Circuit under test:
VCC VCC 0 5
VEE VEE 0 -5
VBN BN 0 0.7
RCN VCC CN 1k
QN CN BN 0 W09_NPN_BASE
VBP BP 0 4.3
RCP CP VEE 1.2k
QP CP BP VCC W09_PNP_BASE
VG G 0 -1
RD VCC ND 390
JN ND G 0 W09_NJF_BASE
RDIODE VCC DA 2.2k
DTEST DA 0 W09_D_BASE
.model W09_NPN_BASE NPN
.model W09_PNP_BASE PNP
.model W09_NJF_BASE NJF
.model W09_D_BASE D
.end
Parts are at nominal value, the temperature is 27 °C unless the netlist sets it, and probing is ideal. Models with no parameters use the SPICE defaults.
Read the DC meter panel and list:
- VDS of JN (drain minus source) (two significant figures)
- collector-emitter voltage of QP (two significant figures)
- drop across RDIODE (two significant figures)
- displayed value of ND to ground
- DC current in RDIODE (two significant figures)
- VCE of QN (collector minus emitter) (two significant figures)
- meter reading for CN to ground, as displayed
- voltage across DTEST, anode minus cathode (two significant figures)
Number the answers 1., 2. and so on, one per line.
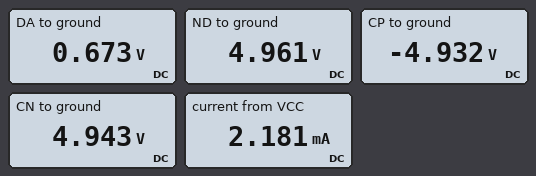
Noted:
1. 5.0 V
2. -9.9 V
3. 4.3 V
4. 4.961 V
5. 2.0 mA
6. 4.9 V
7. 4.943 V
8. 670 mV
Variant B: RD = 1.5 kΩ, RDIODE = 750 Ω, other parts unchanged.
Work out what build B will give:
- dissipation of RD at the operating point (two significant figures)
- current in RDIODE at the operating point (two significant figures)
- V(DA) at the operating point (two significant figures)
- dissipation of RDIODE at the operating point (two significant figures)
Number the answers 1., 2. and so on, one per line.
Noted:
1. 15 µW
2. 5.7 mA
3. 700 mV
4. 25 mW
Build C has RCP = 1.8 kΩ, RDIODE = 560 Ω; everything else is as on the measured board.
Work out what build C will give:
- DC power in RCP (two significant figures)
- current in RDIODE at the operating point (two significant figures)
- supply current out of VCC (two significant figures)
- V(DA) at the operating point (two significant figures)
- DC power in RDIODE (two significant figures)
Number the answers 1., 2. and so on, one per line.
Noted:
1. 5.8 µW
2. 7.7 mA
3. 7.9 mA
4. 710 mV
5. 33 mW
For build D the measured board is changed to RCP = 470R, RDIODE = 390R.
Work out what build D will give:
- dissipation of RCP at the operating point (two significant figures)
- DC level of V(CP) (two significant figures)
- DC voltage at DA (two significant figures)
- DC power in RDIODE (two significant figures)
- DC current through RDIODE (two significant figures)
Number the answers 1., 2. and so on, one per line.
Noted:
1. 1.5 µW
2. -5.0 V
3. 720 mV
4. 47 mW
5. 11 mA
